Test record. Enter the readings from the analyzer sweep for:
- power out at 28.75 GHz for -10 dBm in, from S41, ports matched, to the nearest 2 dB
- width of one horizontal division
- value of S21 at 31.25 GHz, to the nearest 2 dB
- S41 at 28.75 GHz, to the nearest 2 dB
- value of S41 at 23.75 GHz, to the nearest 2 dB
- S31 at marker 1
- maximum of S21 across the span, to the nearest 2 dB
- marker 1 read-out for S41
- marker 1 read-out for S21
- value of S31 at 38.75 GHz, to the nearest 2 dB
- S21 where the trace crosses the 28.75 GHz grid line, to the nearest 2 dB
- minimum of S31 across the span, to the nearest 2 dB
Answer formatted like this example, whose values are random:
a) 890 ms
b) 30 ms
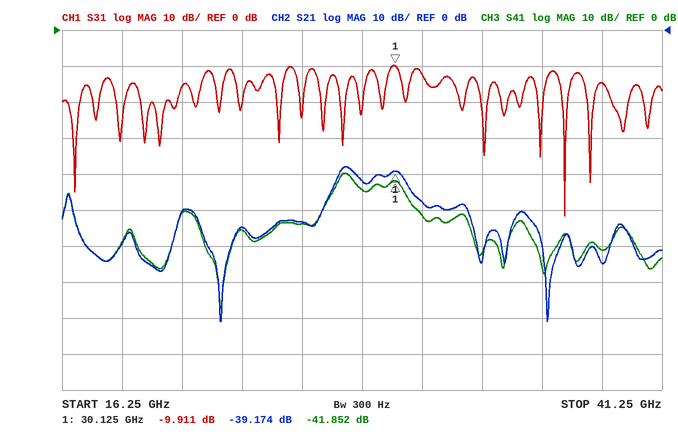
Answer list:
a) -54 dBm
b) 2.5 GHz
c) -48 dB
d) -44 dB
e) -56 dB
f) -9.911 dB
g) -38 dB
h) -41.852 dB
i) -39.174 dB
j) -14 dB
k) -42 dB
l) -52 dB
